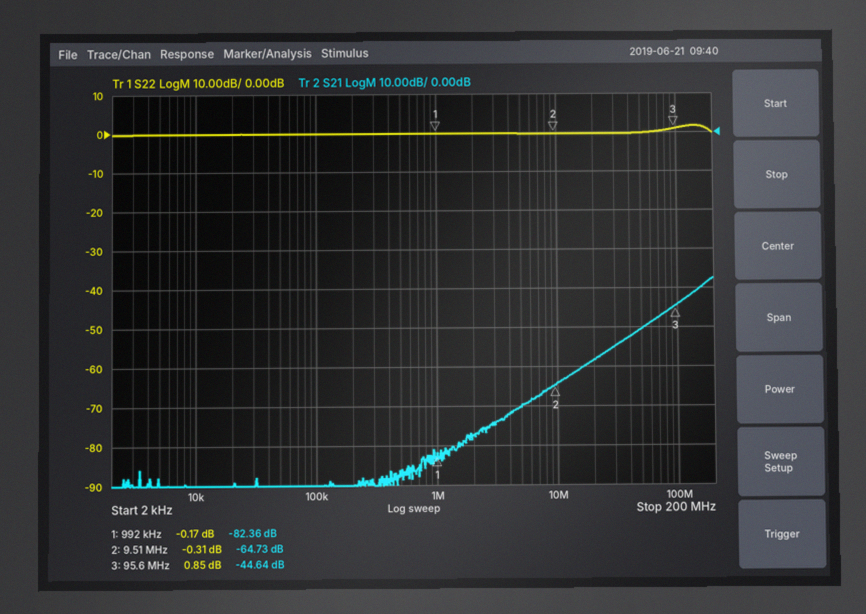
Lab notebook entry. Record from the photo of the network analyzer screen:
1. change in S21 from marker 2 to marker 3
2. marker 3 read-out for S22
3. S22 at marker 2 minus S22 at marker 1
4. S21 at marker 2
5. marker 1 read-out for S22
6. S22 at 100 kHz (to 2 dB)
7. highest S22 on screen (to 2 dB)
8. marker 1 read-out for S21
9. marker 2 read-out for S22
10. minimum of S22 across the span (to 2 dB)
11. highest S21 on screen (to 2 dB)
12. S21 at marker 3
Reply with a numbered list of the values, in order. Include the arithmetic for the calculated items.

1. -44.64 − (-64.73) = 20.09 dB
2. 0.85 dB
3. -0.31 − (-0.17) = -0.14 dB
4. -64.73 dB
5. -0.17 dB
6. 0 dB
7. 2 dB
8. -82.36 dB
9. -0.31 dB
10. 0 dB
11. -38 dB
12. -44.64 dB
